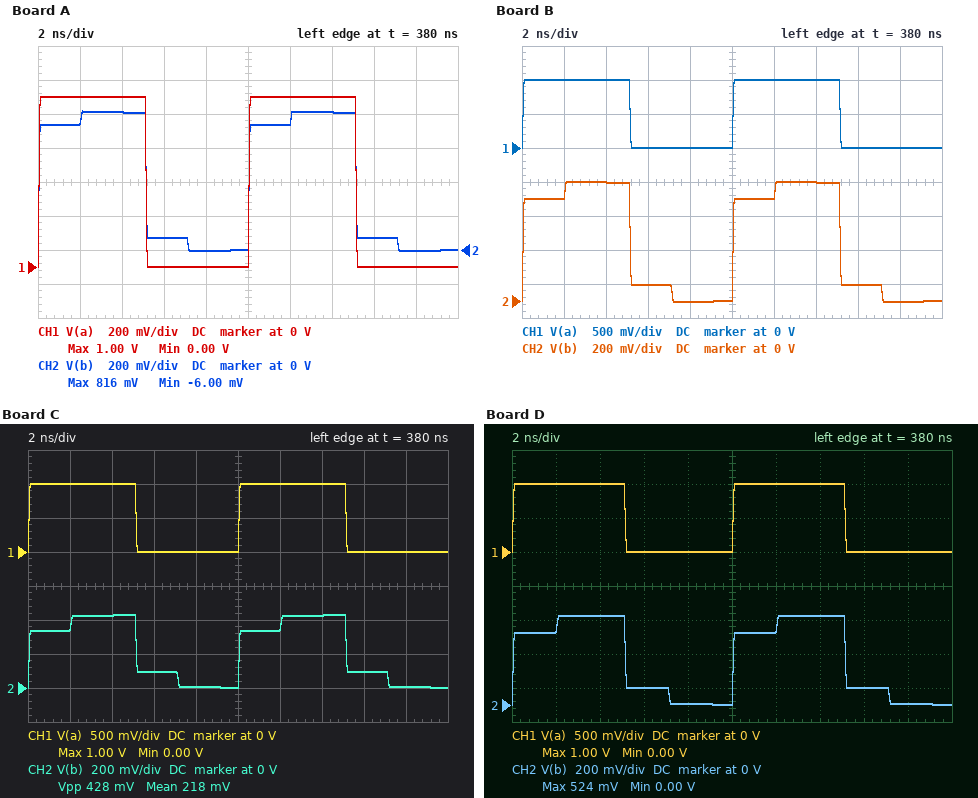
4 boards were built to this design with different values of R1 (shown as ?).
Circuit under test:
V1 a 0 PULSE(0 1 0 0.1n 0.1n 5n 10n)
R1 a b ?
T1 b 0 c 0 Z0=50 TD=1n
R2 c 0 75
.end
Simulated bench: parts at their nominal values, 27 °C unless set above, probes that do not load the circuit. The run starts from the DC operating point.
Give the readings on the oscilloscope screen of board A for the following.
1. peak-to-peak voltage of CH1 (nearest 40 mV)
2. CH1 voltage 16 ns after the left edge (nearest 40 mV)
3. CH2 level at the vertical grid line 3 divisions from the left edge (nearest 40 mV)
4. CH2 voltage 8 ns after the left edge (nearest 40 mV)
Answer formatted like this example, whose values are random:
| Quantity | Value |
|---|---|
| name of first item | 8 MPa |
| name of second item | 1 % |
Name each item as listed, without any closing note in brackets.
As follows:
| Quantity | Value |
|---|---|
| peak-to-peak voltage of CH1 | 1.00 V |
| CH1 voltage 16 ns after the left edge | 0 V |
| CH2 level at the vertical grid line 3 divisions from the left edge | 80 mV |
| CH2 voltage 8 ns after the left edge | 0 V |
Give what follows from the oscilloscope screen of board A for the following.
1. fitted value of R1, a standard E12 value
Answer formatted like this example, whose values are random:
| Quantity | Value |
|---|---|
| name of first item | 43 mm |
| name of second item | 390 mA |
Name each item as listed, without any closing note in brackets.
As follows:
| Quantity | Value |
|---|---|
| fitted value of R1, a standard E12 value | 18 Ω |
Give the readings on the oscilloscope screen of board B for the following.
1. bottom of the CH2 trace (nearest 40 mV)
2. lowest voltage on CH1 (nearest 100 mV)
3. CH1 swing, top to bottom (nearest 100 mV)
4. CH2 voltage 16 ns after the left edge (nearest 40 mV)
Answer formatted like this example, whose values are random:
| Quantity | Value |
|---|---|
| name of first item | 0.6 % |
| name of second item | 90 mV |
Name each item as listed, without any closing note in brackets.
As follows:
| Quantity | Value |
|---|---|
| bottom of the CH2 trace | 0 V |
| lowest voltage on CH1 | 0 V |
| CH1 swing, top to bottom | 1.0 V |
| CH2 voltage 16 ns after the left edge | 80 mV |
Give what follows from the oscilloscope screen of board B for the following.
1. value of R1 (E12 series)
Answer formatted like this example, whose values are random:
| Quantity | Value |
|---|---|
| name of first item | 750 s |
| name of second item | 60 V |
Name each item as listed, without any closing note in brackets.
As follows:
| Quantity | Value |
|---|---|
| value of R1 | 33 Ω |
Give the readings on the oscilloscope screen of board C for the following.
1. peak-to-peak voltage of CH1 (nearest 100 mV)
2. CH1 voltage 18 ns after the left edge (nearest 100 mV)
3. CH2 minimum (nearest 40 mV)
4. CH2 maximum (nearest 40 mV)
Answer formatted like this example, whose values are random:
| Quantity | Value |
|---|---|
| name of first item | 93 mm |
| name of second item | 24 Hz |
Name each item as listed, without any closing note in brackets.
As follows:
| Quantity | Value |
|---|---|
| peak-to-peak voltage of CH1 | 1.0 V |
| CH1 voltage 18 ns after the left edge | 0 V |
| CH2 minimum | 0 V |
| CH2 maximum | 440 mV |
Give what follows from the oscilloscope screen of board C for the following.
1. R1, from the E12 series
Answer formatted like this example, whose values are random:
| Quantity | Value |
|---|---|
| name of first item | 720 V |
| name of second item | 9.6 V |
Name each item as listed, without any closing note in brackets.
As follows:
| Quantity | Value |
|---|---|
| R1, from the E12 series | 100 Ω |
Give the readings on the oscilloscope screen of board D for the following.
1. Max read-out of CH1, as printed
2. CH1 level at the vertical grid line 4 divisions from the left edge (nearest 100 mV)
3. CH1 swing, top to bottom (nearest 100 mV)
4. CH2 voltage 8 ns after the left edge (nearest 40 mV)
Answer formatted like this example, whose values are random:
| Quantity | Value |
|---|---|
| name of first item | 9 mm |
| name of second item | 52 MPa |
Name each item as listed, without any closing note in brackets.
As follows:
| Quantity | Value |
|---|---|
| Max read-out of CH1, as printed | 1.00 V |
| CH1 level at the vertical grid line 4 divisions from the left edge | 0 V |
| CH1 swing, top to bottom | 1.0 V |
| CH2 voltage 8 ns after the left edge | 0 V |
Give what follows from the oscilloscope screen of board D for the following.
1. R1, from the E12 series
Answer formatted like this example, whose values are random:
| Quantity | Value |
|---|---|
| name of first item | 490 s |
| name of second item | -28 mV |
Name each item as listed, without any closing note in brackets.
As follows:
| Quantity | Value |
|---|---|
| R1, from the E12 series | 68 Ω |
